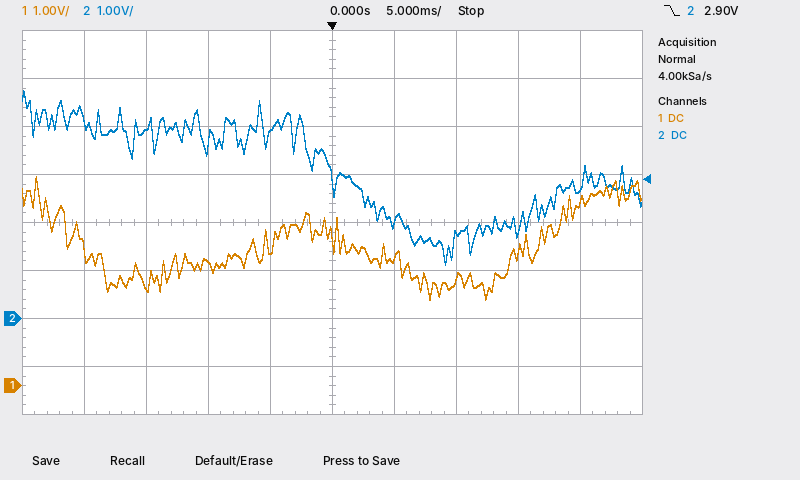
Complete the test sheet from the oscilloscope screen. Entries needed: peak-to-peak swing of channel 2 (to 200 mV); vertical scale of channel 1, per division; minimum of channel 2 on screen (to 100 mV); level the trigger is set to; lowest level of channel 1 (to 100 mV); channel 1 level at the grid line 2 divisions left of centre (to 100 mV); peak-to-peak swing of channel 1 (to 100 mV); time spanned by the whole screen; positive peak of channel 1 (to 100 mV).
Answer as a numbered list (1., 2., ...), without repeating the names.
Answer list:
1. 3.6 V
2. 1 V
3. 1.1 V
4. 2.90 V
5. 1.8 V
6. 2.6 V
7. 2.6 V
8. 50 ms
9. 4.4 V
